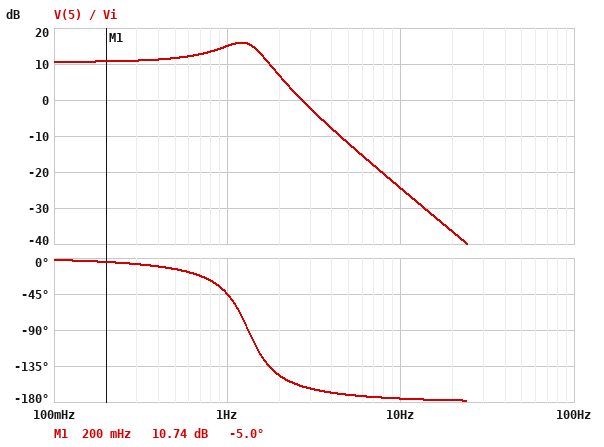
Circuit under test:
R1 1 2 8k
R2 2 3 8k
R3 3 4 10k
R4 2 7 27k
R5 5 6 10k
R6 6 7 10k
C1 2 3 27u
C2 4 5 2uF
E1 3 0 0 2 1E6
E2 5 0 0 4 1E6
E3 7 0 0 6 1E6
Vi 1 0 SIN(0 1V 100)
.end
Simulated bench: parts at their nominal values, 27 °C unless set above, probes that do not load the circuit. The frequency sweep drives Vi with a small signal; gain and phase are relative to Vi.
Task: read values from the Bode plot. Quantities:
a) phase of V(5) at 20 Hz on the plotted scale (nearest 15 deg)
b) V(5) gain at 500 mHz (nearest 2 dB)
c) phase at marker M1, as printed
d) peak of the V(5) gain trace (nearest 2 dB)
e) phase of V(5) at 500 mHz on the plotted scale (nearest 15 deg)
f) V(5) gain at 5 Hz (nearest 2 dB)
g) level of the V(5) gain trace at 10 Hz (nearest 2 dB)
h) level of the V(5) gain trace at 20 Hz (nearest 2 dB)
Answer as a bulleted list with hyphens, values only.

- -180 deg
- 12 dB
- -5.0 deg
- 16 dB
- -15 deg
- -12 dB
- -24 dB
- -36 dB
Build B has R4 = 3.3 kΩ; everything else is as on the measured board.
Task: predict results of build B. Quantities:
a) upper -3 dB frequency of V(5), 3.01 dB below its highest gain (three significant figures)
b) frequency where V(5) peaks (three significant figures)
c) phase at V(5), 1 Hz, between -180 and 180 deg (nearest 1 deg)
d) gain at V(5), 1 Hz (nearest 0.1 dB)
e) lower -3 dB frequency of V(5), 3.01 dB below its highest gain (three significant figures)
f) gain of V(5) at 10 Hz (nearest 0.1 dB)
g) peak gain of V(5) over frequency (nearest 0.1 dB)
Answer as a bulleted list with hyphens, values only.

- 4.09 Hz
- 3.73 Hz
- -3 deg
- -7.1 dB
- 3.34 Hz
- -23.3 dB
- 6.5 dB
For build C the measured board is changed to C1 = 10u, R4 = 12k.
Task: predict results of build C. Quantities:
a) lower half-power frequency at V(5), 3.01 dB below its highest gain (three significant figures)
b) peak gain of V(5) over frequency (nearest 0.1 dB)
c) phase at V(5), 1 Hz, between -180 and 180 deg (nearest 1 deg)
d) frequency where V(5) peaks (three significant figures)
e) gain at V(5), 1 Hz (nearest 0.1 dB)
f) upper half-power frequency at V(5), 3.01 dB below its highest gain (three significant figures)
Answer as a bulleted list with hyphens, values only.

- 1.56 Hz
- 8.2 dB
- -12 deg
- 2.93 Hz
- 4.2 dB
- 3.84 Hz
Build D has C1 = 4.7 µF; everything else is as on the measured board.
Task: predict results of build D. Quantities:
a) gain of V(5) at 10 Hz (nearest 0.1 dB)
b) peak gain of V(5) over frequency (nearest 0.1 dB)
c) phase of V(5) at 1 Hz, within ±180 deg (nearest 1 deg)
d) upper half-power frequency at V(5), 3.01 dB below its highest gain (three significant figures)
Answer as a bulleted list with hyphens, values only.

- -9.4 dB
- 10.6 dB
- -25 deg
- 3.31 Hz
